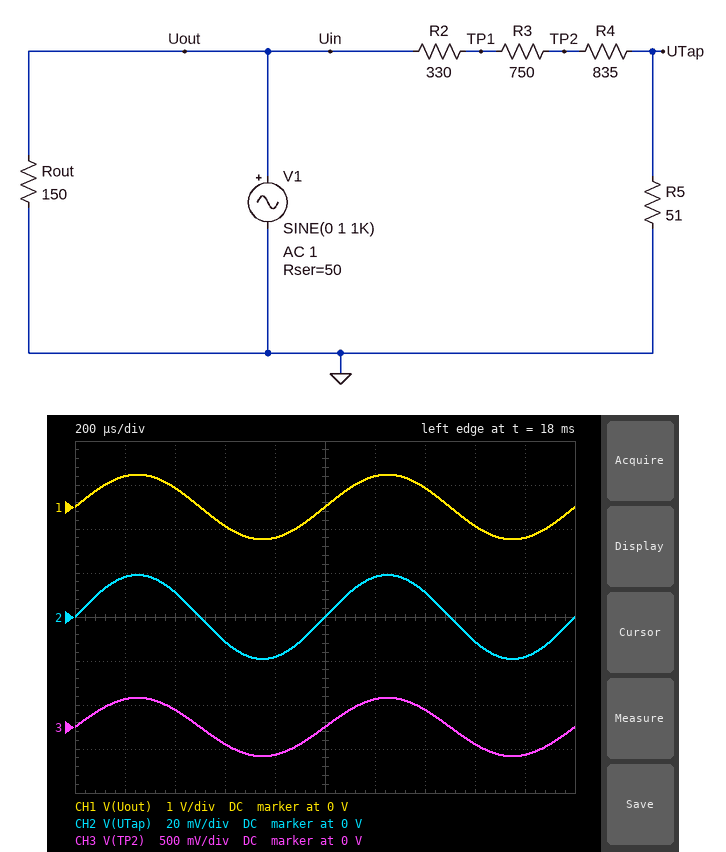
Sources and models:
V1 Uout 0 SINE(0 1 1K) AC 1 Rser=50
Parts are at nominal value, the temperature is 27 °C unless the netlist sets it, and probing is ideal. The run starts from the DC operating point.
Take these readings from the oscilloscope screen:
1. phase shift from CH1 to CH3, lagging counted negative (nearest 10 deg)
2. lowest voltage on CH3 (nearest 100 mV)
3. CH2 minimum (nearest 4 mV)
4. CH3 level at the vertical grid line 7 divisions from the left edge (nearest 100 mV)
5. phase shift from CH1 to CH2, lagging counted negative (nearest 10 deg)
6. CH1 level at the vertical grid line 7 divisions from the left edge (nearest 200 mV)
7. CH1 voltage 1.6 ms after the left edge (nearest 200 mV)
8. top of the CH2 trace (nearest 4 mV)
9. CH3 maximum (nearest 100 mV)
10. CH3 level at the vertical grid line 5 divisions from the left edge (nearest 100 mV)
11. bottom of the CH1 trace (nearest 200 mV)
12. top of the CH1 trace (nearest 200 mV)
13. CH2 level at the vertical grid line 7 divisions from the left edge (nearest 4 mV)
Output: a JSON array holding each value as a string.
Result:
["0 deg", "-300 mV", "-20 mV", "200 mV", "0 deg", "400 mV", "-400 mV", "20 mV", "300 mV", "0 V", "-800 mV", "800 mV", "12 mV"]
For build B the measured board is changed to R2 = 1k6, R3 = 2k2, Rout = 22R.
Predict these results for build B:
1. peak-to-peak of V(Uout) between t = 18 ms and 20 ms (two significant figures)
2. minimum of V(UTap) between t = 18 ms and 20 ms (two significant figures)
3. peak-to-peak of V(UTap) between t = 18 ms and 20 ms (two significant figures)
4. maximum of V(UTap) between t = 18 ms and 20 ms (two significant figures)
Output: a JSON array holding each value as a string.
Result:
["610 mV", "-3.3 mV", "6.6 mV", "3.3 mV"]
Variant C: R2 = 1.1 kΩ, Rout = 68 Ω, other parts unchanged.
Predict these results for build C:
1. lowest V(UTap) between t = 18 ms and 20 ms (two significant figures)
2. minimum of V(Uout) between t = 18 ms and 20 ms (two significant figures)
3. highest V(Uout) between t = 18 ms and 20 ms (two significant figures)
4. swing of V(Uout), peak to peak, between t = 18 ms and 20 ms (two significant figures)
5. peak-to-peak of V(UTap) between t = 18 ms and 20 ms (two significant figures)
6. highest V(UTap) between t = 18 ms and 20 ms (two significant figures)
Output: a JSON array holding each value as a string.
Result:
["-11 mV", "-570 mV", "570 mV", "1.1 V", "21 mV", "11 mV"]
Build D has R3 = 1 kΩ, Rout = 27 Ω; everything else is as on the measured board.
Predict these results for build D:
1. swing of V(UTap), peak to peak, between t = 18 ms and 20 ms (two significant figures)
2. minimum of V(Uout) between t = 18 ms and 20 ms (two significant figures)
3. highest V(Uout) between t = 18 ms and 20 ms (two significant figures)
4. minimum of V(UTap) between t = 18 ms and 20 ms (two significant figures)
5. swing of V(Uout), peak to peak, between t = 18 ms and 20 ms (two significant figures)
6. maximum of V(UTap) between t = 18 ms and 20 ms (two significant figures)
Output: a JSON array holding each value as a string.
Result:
["16 mV", "-350 mV", "350 mV", "-8.0 mV", "700 mV", "8.0 mV"]
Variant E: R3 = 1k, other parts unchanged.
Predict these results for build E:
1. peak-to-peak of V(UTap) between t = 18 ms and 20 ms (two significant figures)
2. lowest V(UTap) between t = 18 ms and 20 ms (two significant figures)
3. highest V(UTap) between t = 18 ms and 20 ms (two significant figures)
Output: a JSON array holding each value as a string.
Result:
["34 mV", "-17 mV", "17 mV"]
